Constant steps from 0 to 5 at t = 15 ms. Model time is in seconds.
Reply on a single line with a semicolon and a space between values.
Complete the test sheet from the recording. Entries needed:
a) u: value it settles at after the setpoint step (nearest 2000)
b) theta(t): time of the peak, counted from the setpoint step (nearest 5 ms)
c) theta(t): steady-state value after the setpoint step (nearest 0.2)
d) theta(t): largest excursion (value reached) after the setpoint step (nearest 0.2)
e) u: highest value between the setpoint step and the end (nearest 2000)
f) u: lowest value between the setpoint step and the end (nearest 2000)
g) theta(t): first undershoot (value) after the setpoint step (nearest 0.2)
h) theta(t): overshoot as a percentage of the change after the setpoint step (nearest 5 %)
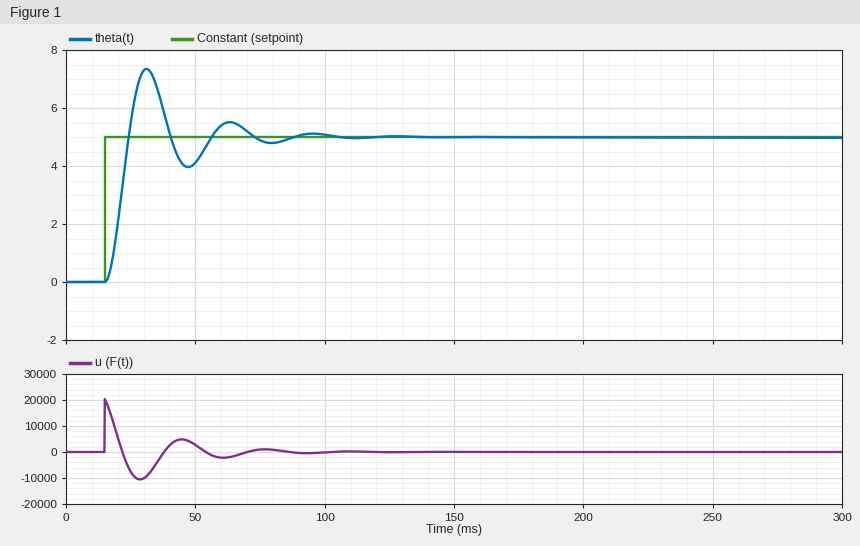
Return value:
0; 15 ms; 5.0; 7.4; 20000; -10000; 4.0; 50 %
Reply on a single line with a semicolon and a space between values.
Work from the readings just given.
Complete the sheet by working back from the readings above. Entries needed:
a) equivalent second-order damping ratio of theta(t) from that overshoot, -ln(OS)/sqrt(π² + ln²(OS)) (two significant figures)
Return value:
0.22
